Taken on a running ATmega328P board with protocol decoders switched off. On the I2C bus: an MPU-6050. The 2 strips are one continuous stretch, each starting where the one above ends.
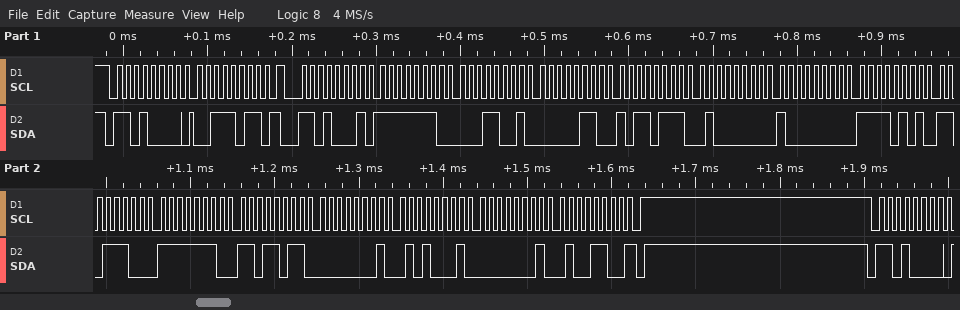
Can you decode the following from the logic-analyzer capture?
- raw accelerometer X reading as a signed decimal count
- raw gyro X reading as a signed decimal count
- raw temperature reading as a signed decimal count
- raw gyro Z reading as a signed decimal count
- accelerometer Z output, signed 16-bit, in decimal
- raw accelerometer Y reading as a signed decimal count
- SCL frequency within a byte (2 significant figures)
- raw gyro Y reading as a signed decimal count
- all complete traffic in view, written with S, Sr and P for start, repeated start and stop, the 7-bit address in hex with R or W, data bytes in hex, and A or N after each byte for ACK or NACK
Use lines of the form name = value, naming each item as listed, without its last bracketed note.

raw accelerometer X reading as a signed decimal count = -487
raw gyro X reading as a signed decimal count = -293
raw temperature reading as a signed decimal count = -2596
raw gyro Z reading as a signed decimal count = 332
accelerometer Z output, signed 16-bit, in decimal = 16512
raw accelerometer Y reading as a signed decimal count = 1719
SCL frequency within a byte = 100 kHz
raw gyro Y reading as a signed decimal count = 337
all complete traffic in view, written with S, Sr and P for start, repeated start and stop, the 7-bit address in hex with R or W, data bytes in hex, and A or N after each byte for ACK or NACK = S 68W A 3B A Sr 68R A FE A 19 A 06 A B7 A 40 A 80 A F5 A DC A FE A DB A 01 A 51 A 01 A 4C N P S 68W A
